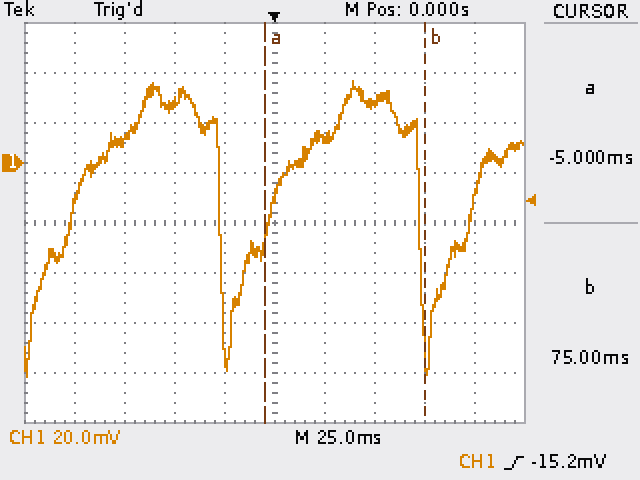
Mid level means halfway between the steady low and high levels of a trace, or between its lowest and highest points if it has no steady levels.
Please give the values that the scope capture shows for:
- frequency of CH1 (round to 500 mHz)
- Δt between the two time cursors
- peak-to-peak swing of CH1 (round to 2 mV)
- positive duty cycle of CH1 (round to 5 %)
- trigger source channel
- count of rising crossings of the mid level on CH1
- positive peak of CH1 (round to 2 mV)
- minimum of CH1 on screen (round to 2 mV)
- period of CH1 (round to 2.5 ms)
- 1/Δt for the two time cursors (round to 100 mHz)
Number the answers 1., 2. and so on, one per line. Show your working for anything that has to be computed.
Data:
1. 1 / 100.0 ms ≈ 10.0 Hz
2. 75 ms − (-5 ms) = 80.0 ms
3. 32 mV − (-86 mV) = 118 mV
4. 75 %
5. CH1
6. 3
7. 32 mV
8. -86 mV
9. 100.0 ms
10. 1 / 80.0 ms ≈ 12.5 Hz
